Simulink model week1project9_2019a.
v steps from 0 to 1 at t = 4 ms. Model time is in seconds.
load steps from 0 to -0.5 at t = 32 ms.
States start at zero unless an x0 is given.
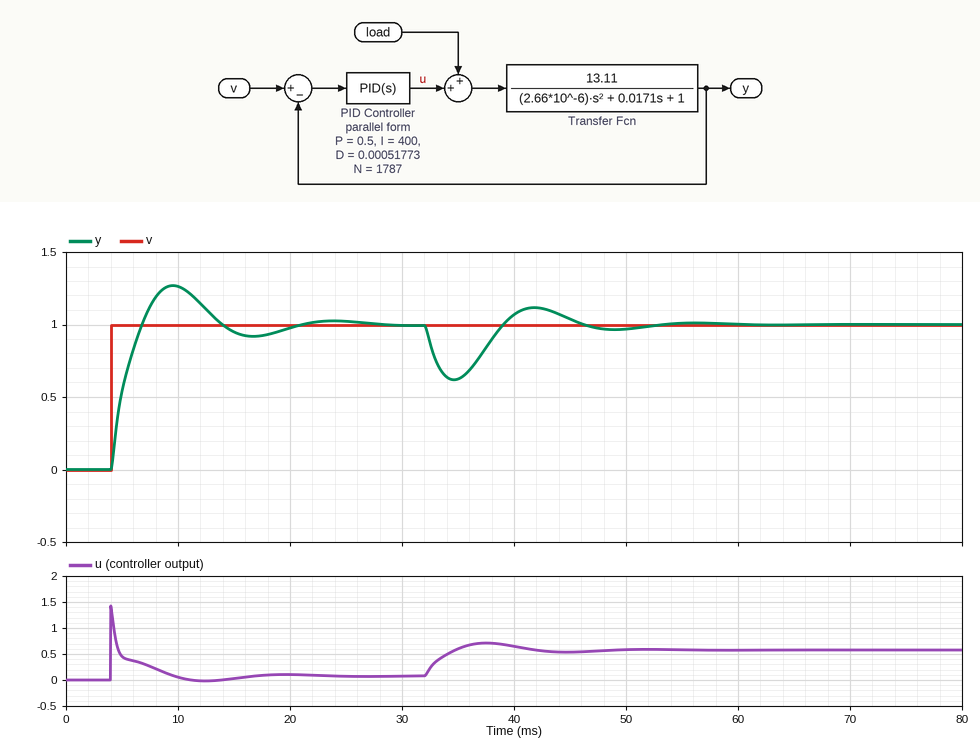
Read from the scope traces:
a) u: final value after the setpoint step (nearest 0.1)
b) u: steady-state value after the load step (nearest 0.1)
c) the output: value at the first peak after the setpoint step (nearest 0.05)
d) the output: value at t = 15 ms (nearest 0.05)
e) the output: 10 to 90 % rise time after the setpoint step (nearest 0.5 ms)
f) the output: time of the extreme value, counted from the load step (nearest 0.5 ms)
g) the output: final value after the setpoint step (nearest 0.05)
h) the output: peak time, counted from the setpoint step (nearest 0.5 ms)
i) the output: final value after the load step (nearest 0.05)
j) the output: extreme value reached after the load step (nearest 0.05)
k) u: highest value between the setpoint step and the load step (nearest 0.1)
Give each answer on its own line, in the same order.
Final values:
0.1
0.6
1.25
0.95
2.0 ms
2.5 ms
1.00
5.5 ms
1.00
0.60
1.4
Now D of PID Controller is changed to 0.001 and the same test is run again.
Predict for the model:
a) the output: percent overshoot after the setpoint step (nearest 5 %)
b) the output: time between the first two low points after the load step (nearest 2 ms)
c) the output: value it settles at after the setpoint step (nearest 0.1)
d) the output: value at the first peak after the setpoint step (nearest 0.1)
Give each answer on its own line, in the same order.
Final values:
20 %
16 ms
1.0
1.2
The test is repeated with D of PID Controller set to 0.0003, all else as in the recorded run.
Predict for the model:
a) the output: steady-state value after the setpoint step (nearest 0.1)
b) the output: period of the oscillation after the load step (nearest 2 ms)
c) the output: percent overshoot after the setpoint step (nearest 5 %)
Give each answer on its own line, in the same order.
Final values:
1.0
14 ms
30 %
